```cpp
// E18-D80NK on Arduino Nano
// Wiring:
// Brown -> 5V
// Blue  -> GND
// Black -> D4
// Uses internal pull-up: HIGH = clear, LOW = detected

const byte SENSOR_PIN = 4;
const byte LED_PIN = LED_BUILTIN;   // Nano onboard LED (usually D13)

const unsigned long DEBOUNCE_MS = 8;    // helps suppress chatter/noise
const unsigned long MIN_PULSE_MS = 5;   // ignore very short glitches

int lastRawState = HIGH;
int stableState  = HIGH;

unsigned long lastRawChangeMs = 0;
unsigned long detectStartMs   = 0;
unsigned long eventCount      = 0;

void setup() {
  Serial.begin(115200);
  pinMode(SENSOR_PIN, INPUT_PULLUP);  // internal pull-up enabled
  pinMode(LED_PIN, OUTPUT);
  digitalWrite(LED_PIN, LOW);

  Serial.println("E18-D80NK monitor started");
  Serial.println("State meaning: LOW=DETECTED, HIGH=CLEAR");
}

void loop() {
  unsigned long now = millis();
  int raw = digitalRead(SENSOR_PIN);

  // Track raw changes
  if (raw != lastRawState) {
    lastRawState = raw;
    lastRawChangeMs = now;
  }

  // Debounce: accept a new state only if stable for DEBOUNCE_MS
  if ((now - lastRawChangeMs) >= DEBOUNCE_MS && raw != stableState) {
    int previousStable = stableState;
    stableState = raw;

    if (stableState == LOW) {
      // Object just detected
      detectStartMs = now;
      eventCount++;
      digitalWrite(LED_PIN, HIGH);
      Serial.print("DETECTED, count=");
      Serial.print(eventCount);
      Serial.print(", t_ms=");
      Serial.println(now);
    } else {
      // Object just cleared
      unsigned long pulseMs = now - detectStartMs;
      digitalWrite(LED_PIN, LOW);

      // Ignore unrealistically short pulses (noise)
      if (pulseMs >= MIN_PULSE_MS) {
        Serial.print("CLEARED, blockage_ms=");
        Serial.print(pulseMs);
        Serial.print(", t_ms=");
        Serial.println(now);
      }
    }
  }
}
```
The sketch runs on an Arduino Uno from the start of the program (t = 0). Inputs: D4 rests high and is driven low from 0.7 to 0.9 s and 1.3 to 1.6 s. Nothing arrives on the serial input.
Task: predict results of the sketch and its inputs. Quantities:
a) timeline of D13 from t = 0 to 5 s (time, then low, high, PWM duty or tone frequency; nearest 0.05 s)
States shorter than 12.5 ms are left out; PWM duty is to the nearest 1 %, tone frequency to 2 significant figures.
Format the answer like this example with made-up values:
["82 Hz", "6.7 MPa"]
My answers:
["0 s low; 0.7 s high; 0.9 s low; 1.3 s high; 1.6 s low"]
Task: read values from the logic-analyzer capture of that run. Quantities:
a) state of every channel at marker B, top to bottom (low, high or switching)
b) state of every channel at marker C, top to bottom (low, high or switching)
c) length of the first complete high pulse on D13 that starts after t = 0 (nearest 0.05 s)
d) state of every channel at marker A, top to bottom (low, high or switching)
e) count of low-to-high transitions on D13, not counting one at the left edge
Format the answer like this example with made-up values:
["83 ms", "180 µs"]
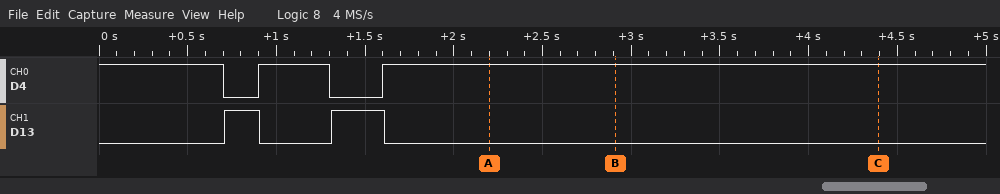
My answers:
["D4 high, D13 low", "D4 high, D13 low", "0.20 s", "D4 high, D13 low", "2"]
